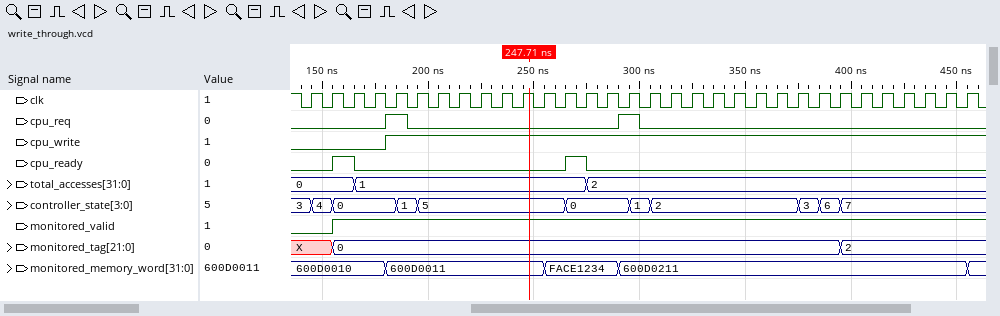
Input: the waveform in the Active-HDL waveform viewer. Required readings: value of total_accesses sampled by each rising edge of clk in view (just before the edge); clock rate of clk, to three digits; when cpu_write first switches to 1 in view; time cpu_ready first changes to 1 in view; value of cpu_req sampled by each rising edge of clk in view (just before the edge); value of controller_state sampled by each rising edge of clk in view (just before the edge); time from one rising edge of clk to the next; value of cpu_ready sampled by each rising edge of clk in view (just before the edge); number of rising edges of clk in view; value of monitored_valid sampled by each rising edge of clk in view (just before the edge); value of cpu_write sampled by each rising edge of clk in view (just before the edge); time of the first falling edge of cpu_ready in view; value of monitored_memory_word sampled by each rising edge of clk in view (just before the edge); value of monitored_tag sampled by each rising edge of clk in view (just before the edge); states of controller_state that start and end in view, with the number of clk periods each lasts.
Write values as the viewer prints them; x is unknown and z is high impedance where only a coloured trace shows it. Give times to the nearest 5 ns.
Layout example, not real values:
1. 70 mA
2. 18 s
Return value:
1. 0, 0, 0, 1, 1, 1, 1, 1, 1, 1, 1, 1, 1, 1, 2, 2, 2, 2, 2, 2, 2, 2, 2, 2, 2, 2, 2, 2, 2, 2, 2, 2
2. 100 MHz
3. 180 ns
4. 155 ns
5. 0 0 0 0 1 0 0 0 0 0 0 0 0 0 0 1 0 0 0 0 0 0 0 0 0 0 0 0 0 0 0 0
6. 3, 4, 0, 0, 0, 1, 5, 5, 5, 5, 5, 5, 5, 0, 0, 0, 1, 2, 2, 2, 2, 2, 2, 2, 3, 6, 7, 7, 7, 7, 7, 7
7. 10 ns
8. 0 0 1 0 0 0 0 0 0 0 0 0 0 1 0 0 0 0 0 0 0 0 0 0 0 0 0 0 0 0 0 0
9. 32
10. 0 0 1 1 1 1 1 1 1 1 1 1 1 1 1 1 1 1 1 1 1 1 1 1 1 1 1 1 1 1 1 1
11. 0 0 0 0 1 1 1 1 1 1 1 1 1 1 1 1 1 1 1 1 1 1 1 1 1 1 1 1 1 1 1 1
12. 165 ns
13. 600D0010, 600D0010, 600D0010, 600D0010, 600D0011, 600D0011, 600D0011, 600D0011, 600D0011, 600D0011, 600D0011, 600D0011, FACE1234, FACE1234, FACE1234, 600D0211, 600D0211, 600D0211, 600D0211, 600D0211, 600D0211, 600D0211, 600D0211, 600D0211, 600D0211, 600D0211, 600D0211, 600D0211, 600D0211, 600D0211, 600D0211, 600D0211
14. X, X, 0, 0, 0, 0, 0, 0, 0, 0, 0, 0, 0, 0, 0, 0, 0, 0, 0, 0, 0, 0, 0, 0, 0, 0, 2, 2, 2, 2, 2, 2
15. 4: 1, 0: 3, 1: 1, 5: 7, 0: 3, 1: 1, 2: 7, 3: 1, 6: 1
